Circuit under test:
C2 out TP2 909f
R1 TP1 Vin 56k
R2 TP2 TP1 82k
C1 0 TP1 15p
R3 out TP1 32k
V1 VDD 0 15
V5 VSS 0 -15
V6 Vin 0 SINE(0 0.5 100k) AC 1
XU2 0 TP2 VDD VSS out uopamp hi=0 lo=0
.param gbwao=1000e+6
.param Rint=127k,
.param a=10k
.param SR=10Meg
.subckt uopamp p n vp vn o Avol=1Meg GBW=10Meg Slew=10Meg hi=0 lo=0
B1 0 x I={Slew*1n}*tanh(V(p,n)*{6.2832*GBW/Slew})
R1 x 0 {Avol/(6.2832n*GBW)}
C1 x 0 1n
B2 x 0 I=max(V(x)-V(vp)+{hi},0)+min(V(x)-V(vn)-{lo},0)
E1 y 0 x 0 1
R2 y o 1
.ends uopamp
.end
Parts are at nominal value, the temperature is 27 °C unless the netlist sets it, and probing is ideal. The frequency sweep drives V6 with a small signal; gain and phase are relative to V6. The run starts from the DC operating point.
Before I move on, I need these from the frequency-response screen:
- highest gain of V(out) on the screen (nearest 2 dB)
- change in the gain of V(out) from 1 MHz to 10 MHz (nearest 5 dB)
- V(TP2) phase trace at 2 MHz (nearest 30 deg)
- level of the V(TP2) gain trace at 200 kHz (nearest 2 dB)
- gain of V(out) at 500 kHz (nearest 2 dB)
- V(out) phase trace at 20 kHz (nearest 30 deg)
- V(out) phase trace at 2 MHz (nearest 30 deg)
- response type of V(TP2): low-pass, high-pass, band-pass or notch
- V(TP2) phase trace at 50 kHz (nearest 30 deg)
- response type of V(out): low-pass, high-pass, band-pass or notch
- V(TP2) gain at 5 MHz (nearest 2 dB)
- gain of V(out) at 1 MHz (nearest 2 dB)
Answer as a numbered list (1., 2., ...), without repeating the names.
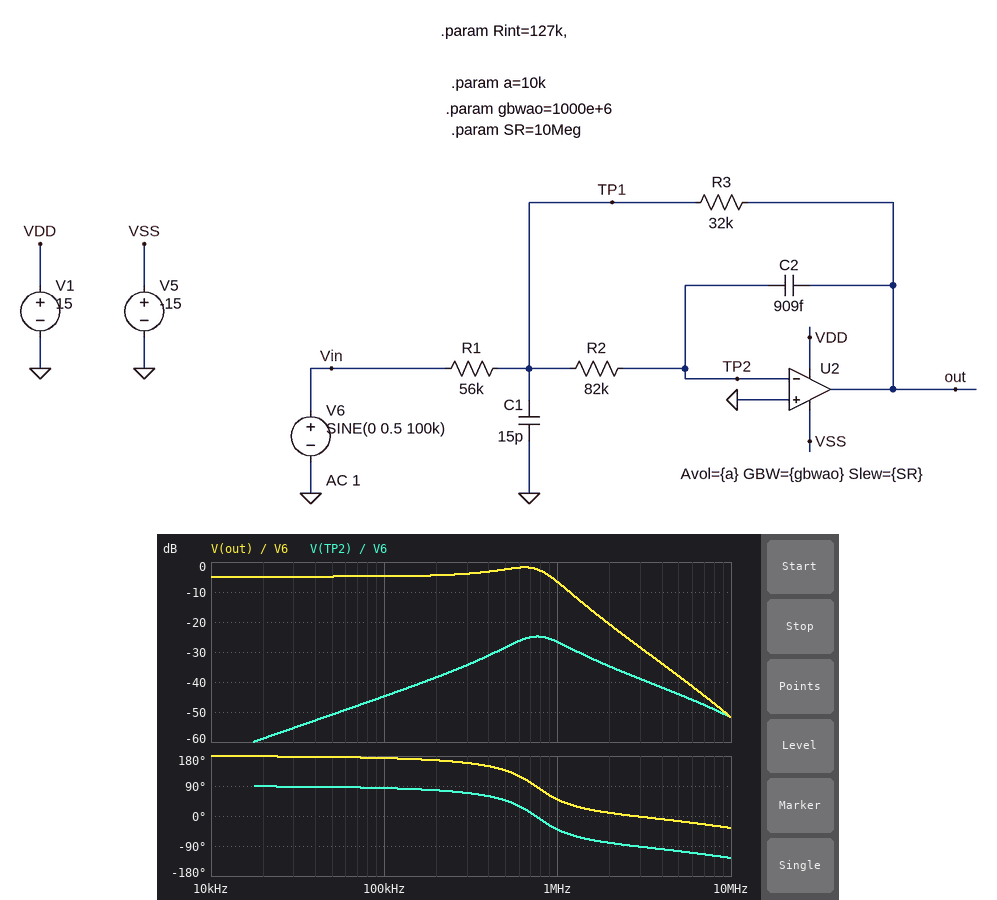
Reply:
1. -2 dB
2. -45 dB
3. -90 deg
4. -38 dB
5. -2 dB
6. 180 deg
7. 0 deg
8. band-pass
9. 90 deg
10. low-pass
11. -44 dB
12. -6 dB
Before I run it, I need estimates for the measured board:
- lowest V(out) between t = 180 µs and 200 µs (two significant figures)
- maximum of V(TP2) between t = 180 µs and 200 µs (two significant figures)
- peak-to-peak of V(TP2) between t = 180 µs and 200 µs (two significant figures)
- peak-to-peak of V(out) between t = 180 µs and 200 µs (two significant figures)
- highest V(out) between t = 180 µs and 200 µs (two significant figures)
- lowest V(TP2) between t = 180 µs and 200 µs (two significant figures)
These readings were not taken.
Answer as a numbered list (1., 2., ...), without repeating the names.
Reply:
1. -290 mV
2. 2.9 mV
3. 5.8 mV
4. 580 mV
5. 290 mV
6. -2.9 mV
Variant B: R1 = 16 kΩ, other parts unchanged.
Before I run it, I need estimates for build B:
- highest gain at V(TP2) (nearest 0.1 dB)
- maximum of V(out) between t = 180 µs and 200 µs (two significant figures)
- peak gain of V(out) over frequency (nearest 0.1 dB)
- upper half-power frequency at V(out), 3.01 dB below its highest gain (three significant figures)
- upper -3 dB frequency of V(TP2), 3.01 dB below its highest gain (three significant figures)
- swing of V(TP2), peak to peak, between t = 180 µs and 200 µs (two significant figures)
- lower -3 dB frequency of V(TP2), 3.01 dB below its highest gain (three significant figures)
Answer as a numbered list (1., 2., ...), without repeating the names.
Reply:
1. -19.1 dB
2. 1.0 V
3. 6.0 dB
4. 780 kHz
5. 1.44 MHz
6. 20 mV
7. 400 kHz
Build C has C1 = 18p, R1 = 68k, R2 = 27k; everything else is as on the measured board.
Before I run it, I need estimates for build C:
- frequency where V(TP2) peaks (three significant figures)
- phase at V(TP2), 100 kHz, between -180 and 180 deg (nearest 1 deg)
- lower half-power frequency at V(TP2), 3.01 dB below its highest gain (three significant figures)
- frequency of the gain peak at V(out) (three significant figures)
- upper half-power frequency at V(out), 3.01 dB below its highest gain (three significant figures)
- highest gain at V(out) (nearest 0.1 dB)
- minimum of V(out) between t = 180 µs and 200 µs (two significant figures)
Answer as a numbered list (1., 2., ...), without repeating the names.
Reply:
1. 1.04 MHz
2. 87 deg
3. 803 kHz
4. 965 kHz
5. 1.21 MHz
6. -0.5 dB
7. -240 mV
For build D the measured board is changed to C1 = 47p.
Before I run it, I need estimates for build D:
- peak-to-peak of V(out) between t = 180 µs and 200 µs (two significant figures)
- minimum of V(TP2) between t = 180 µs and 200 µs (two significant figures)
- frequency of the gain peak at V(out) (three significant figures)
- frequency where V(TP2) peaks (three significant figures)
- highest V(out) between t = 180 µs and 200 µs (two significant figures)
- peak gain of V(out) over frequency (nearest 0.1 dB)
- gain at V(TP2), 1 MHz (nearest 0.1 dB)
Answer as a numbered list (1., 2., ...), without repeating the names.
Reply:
1. 600 mV
2. -3.0 mV
3. 411 kHz
4. 431 kHz
5. 300 mV
6. 2.7 dB
7. -37.9 dB
